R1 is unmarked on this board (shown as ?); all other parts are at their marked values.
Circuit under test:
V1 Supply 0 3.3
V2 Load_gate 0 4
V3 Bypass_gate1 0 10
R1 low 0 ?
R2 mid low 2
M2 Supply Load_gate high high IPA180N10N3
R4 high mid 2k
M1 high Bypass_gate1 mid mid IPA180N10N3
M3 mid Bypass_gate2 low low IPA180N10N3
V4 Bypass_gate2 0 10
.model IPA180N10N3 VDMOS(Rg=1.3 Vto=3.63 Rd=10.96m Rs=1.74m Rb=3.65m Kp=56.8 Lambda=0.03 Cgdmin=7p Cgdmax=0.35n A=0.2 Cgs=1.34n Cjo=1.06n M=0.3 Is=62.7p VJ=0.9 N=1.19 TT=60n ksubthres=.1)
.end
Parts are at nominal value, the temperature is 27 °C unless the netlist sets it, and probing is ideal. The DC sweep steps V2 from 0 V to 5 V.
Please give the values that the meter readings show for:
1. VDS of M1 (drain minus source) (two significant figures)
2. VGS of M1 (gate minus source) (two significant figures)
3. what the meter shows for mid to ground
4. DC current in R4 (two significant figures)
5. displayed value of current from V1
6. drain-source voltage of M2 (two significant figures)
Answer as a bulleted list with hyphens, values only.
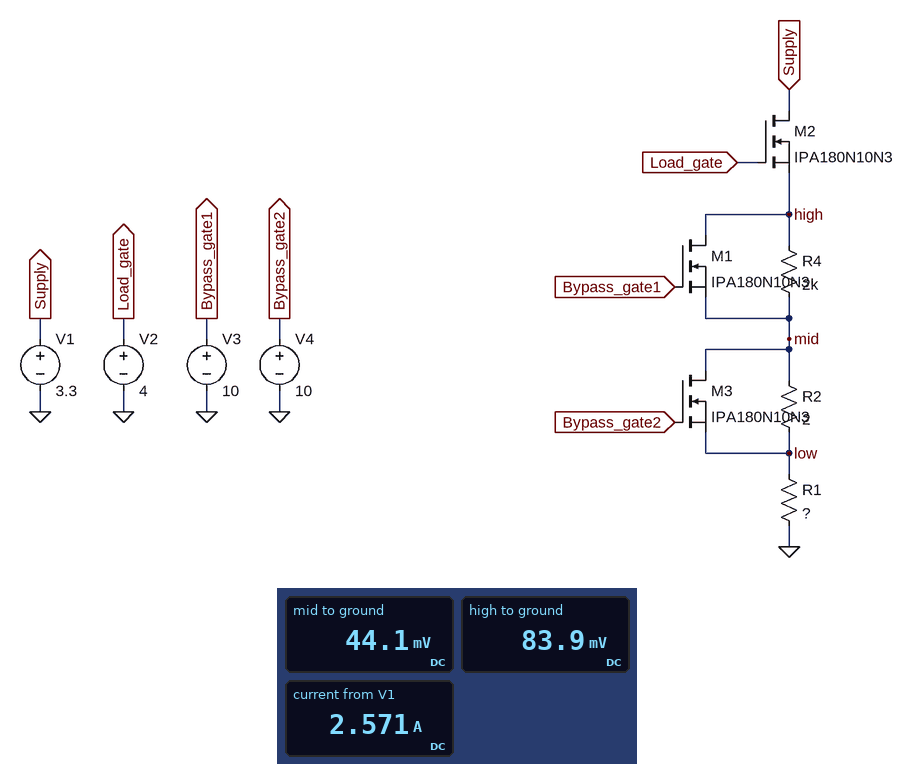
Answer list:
- 40 mV
- 10 V
- 44.1 mV
- 20 µA
- 2.571 A
- 3.2 V
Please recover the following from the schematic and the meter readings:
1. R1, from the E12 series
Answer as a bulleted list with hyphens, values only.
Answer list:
- 1.8 mΩ
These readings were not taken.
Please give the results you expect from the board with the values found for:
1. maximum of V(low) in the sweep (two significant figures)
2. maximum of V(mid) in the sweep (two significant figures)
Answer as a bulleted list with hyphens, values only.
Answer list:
- 32 mV
- 300 mV
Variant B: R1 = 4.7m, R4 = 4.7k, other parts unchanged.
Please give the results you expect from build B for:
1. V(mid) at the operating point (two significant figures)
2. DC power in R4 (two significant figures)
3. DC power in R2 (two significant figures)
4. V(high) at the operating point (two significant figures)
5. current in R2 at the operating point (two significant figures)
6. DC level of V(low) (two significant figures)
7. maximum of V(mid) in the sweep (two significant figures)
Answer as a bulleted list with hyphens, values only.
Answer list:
- 50 mV
- 320 nW
- 730 µW
- 89 mV
- 19 mA
- 12 mV
- 340 mV
